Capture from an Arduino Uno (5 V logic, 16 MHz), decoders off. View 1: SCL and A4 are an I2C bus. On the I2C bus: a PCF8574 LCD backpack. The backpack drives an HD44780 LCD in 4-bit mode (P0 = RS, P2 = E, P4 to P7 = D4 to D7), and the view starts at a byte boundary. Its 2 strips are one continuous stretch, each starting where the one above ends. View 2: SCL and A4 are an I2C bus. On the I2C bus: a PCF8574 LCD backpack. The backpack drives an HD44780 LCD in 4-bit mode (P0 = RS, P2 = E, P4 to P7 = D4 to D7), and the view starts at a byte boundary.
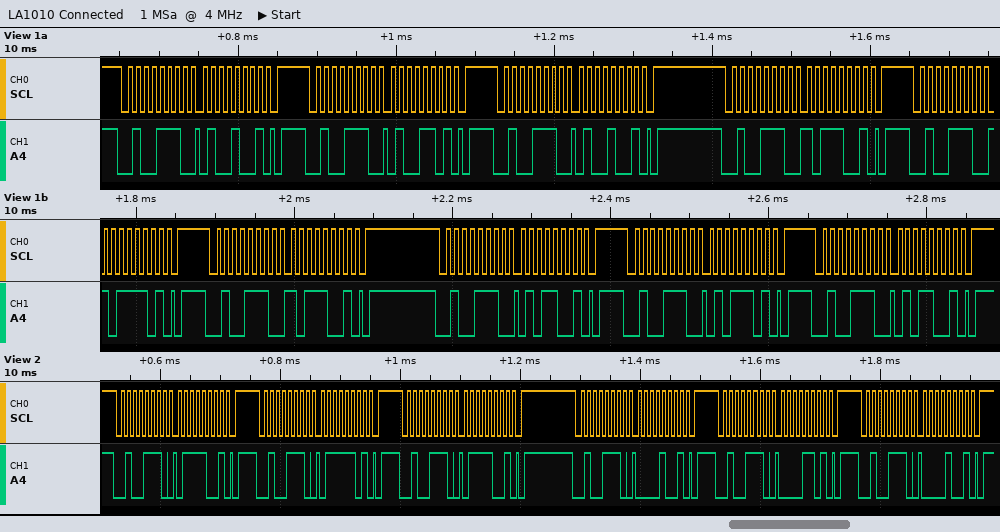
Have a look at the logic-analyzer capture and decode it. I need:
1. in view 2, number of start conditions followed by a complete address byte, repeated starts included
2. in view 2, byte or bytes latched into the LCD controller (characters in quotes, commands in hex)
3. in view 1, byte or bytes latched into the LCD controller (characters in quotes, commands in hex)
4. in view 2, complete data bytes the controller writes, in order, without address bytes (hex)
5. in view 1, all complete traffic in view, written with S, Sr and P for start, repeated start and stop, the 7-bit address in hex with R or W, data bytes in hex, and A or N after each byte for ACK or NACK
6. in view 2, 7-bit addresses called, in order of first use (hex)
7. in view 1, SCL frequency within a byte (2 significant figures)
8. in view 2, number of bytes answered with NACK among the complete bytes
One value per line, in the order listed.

6
'p'
'K'
79 7D 79 09 0D 09
S 27W A 49 A P S 27W A 4D A P S 27W A 49 A P S 27W A B9 A P S 27W A BD A P S 27W A B9 A P S 27W A 59 A P S 27W A 5D A P S 27W A 59 A P
0x27
100 kHz
0
